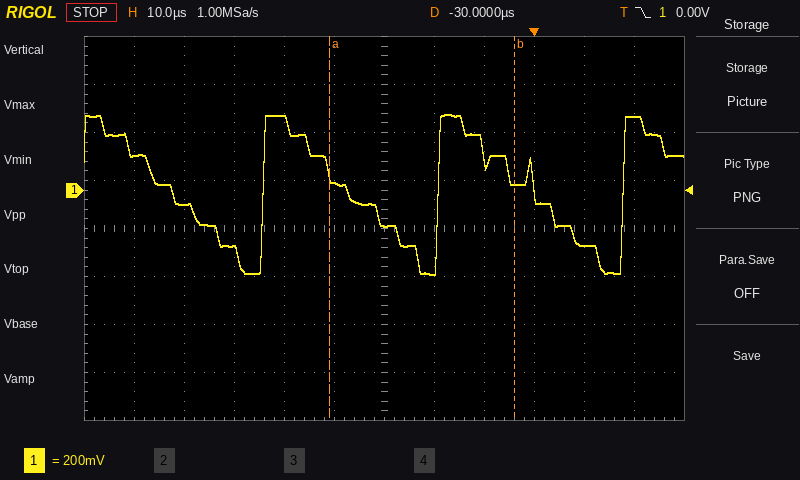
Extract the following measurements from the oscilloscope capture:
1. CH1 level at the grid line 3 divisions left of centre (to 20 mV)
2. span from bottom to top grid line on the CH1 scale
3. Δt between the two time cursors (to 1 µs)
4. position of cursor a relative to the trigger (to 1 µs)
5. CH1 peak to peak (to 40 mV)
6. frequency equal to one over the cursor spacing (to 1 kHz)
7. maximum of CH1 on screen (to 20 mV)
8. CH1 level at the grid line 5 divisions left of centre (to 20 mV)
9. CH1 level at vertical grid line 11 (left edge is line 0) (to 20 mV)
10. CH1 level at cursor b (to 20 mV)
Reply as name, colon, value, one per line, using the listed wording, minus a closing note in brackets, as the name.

CH1 level at the grid line 3 divisions left of centre: -240 mV
span from bottom to top grid line on the CH1 scale: 1.6 V
Δt between the two time cursors: 37 µs
position of cursor a relative to the trigger: -41 µs
CH1 peak to peak: 680 mV
frequency equal to one over the cursor spacing: 27 kHz
maximum of CH1 on screen: 320 mV
CH1 level at the grid line 5 divisions left of centre: 140 mV
CH1 level at vertical grid line 11 (left edge is line 0): 300 mV
CH1 level at cursor b: 20 mV
